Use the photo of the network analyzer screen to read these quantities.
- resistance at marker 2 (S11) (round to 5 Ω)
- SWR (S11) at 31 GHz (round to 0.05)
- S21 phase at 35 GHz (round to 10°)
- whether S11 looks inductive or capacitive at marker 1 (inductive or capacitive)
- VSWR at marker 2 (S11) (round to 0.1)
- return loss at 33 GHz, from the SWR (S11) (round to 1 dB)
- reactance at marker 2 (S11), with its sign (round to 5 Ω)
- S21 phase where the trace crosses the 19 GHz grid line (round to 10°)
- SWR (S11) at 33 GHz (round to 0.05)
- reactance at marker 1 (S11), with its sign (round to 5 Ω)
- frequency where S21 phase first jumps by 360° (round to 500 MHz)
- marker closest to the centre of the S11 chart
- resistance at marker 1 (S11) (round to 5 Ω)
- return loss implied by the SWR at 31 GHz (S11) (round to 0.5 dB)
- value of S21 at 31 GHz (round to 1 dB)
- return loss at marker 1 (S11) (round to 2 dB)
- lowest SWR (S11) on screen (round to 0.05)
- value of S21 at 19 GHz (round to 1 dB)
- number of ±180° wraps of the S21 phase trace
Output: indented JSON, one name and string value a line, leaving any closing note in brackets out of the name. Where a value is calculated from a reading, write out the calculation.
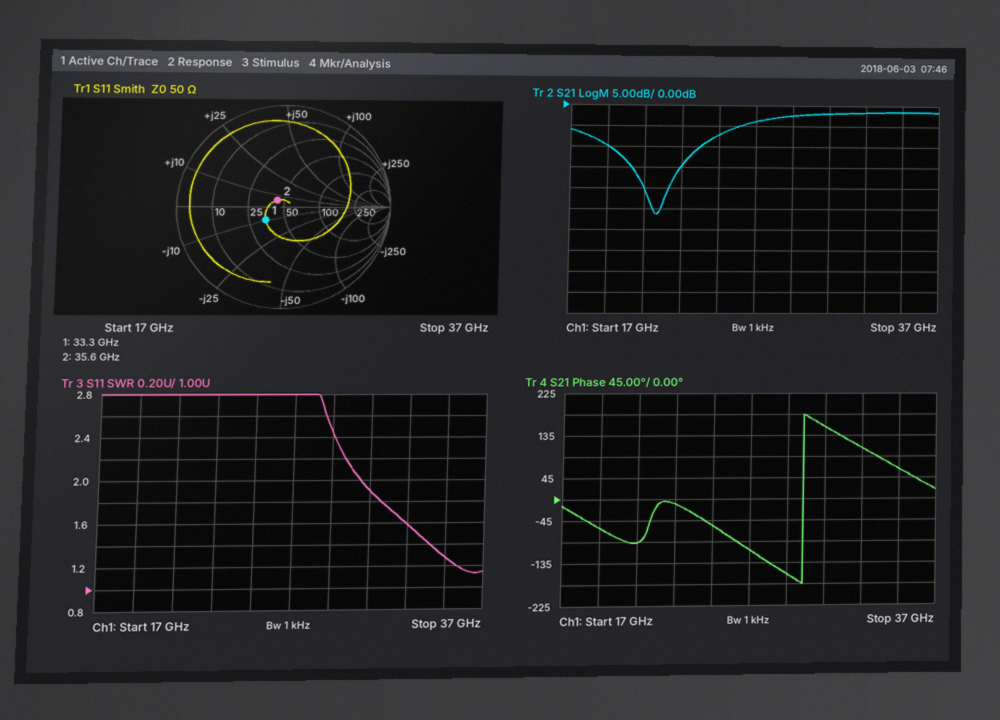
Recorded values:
{
  "resistance at marker 2 (S11)": "45 Ω",
  "SWR (S11) at 31 GHz": "1.90",
  "S21 phase at 35 GHz": "60°",
  "whether S11 looks inductive or capacitive at marker 1": "capacitive",
  "VSWR at marker 2 (S11)": "1.2",
  "return loss at 33 GHz, from the SWR (S11)": "−20 log10((1.6 − 1)/(1.6 + 1)) ≈ 13 dB",
  "reactance at marker 2 (S11), with its sign": "+5 Ω",
  "S21 phase where the trace crosses the 19 GHz grid line": "-60°",
  "SWR (S11) at 33 GHz": "1.60",
  "reactance at marker 1 (S11), with its sign": "-10 Ω",
  "frequency where S21 phase first jumps by 360°": "30.0 GHz",
  "marker closest to the centre of the S11 chart": "marker 2",
  "resistance at marker 1 (S11)": "35 Ω",
  "return loss implied by the SWR at 31 GHz (S11)": "−20 log10((1.9 − 1)/(1.9 + 1)) ≈ 10.2 dB, so 10.0 dB to the nearest 0.5 dB",
  "value of S21 at 31 GHz": "-2 dB",
  "return loss at marker 1 (S11)": "14 dB",
  "lowest SWR (S11) on screen": "1.15",
  "value of S21 at 19 GHz": "-10 dB",
  "number of ±180° wraps of the S21 phase trace": "1"
}
